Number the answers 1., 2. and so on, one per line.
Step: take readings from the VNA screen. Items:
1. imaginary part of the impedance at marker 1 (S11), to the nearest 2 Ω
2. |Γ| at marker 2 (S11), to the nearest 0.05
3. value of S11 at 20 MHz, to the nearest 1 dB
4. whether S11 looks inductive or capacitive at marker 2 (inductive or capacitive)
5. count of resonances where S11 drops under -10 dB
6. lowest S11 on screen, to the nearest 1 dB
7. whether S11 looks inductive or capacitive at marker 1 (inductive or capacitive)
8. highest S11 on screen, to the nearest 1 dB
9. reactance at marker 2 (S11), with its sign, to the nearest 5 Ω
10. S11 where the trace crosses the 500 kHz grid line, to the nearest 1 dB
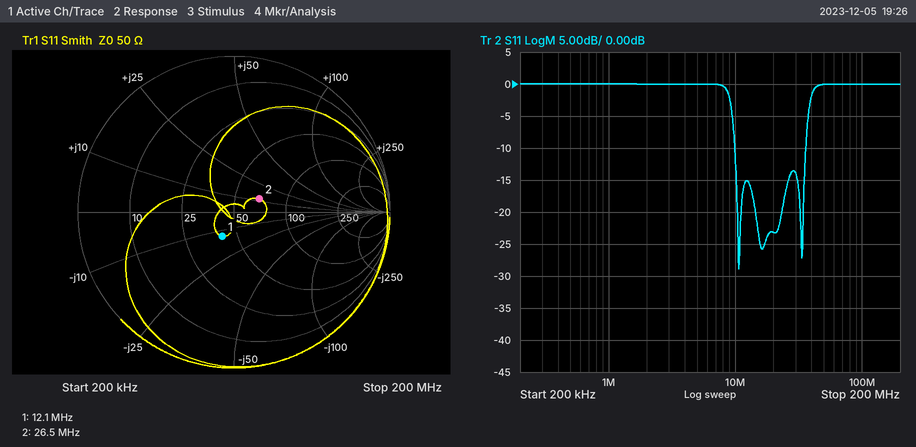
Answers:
1. -14 Ω
2. 0.20
3. -23 dB
4. inductive
5. 3
6. -29 dB
7. capacitive
8. 0 dB
9. +10 Ω
10. 0 dB
